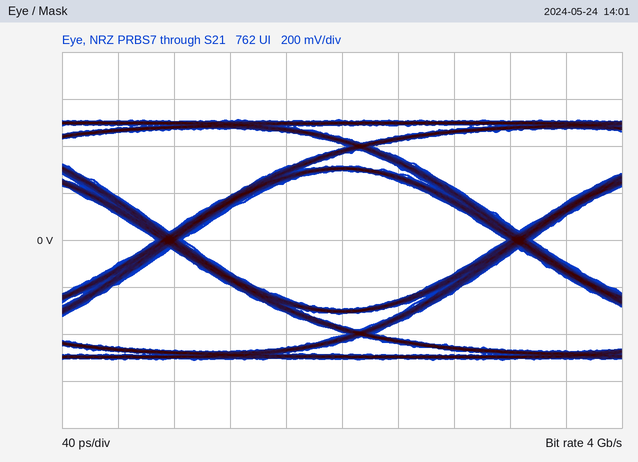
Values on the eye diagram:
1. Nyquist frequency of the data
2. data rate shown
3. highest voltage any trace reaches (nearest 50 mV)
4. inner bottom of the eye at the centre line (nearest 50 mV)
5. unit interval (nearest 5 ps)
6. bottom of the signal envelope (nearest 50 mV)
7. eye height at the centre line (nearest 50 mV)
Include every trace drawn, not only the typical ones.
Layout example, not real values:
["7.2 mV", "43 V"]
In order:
["2 GHz", "4 Gb/s", "500 mV", "-300 mV", "250 ps", "-500 mV", "600 mV"]
